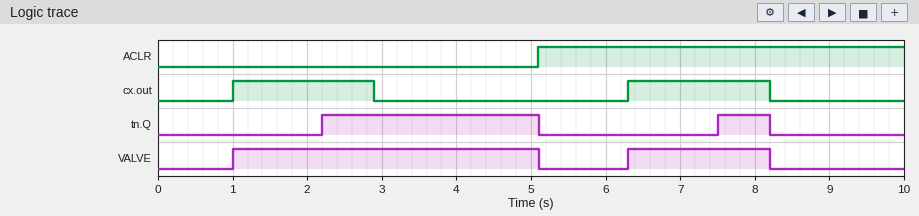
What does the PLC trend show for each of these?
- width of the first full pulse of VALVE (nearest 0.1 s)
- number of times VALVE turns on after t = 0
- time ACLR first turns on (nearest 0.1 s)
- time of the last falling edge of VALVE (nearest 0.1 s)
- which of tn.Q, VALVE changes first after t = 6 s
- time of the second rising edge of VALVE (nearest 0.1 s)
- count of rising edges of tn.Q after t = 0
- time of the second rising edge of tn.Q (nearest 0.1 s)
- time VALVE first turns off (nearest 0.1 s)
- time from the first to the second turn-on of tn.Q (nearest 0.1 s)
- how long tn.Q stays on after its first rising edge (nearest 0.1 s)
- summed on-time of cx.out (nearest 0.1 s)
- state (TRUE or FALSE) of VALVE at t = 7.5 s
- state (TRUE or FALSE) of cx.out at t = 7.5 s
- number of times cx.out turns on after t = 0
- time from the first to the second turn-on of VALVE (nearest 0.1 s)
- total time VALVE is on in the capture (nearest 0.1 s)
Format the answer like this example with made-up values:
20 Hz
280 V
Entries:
4.1 s
2
5.1 s
8.2 s
VALVE
6.3 s
2
7.5 s
5.1 s
5.3 s
2.9 s
3.8 s
TRUE
TRUE
2
5.3 s
6.0 s
